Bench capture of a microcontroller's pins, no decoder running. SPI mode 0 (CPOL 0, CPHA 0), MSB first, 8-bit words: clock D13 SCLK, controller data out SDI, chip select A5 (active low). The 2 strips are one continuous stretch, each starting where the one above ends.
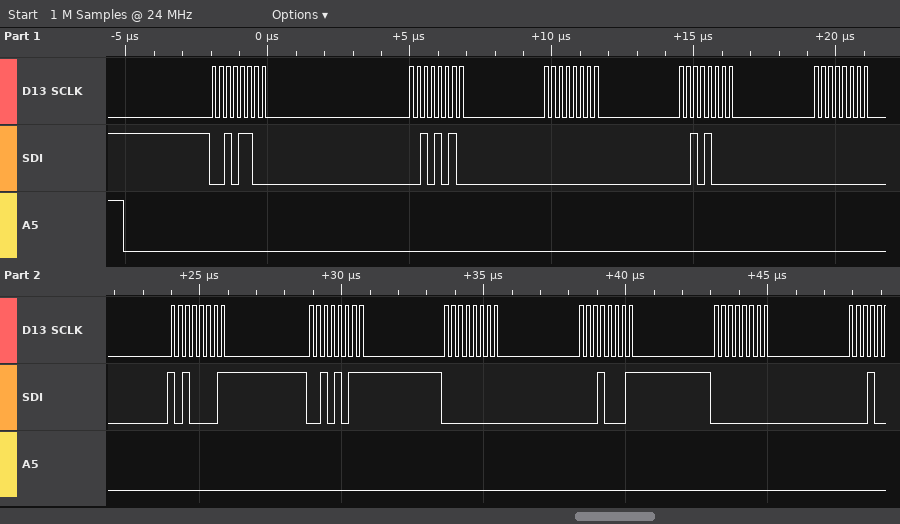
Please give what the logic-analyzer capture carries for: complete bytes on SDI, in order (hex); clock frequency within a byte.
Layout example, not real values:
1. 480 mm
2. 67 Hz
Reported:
1. 2C 2A 00 28 00 A1 2B 00 11 00
2. 4 MHz
